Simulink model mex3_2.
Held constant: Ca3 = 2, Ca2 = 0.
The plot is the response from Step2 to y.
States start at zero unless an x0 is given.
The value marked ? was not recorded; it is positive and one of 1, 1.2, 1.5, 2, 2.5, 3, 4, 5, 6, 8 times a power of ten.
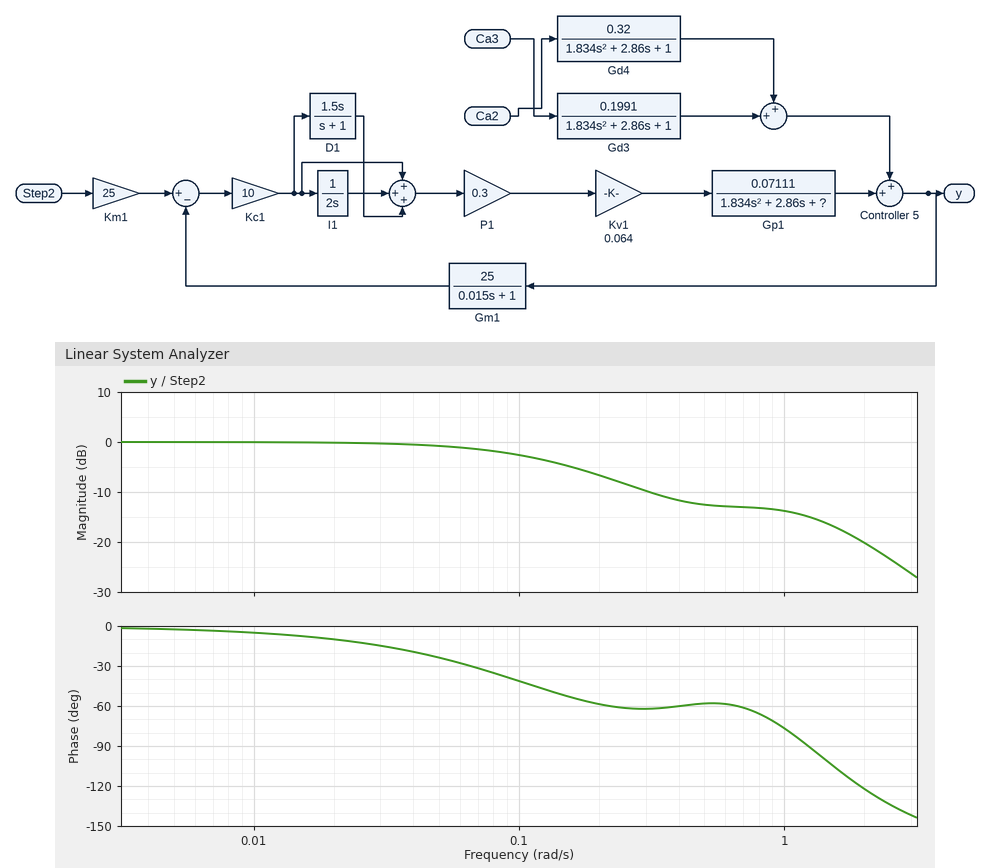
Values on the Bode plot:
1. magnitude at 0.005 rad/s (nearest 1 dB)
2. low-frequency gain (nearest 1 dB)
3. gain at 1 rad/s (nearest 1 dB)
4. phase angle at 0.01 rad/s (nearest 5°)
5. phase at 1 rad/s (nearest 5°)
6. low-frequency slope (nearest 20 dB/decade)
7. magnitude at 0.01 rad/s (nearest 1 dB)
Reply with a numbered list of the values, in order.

1. 0 dB
2. 0 dB
3. -14 dB
4. -5°
5. -75°
6. 0 dB/decade
7. 0 dB
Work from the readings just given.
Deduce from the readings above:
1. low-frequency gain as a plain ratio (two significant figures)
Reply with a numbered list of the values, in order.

1. 1.0
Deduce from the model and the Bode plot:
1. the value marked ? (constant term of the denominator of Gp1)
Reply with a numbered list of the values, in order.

1. 1.5
